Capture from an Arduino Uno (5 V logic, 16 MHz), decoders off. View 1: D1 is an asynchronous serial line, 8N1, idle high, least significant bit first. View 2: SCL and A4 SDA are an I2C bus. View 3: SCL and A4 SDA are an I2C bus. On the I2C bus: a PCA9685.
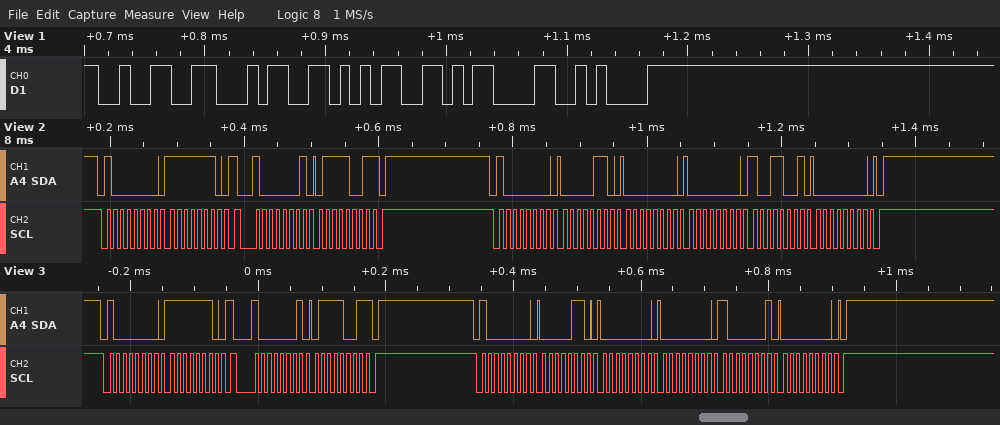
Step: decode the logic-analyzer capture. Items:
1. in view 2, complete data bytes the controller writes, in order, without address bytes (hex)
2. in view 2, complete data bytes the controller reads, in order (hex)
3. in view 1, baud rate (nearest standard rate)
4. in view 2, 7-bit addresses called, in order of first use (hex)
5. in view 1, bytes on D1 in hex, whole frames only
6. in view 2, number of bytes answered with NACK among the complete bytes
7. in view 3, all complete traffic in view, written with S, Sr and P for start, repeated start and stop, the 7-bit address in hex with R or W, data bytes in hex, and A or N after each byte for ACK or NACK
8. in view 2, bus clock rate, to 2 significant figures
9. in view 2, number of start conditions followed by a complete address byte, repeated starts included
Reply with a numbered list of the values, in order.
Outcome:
1. FE 06 00 00 99 00
2. 79
3. 115200 baud
4. 0x40
5. 0x32 0x34 0x35 0x0D 0x0A
6. 1
7. S 40W A FE A Sr 40R A 79 N P S 40W A 06 A 00 A 00 A 81 A 00 A P
8. 100 kHz
9. 3
